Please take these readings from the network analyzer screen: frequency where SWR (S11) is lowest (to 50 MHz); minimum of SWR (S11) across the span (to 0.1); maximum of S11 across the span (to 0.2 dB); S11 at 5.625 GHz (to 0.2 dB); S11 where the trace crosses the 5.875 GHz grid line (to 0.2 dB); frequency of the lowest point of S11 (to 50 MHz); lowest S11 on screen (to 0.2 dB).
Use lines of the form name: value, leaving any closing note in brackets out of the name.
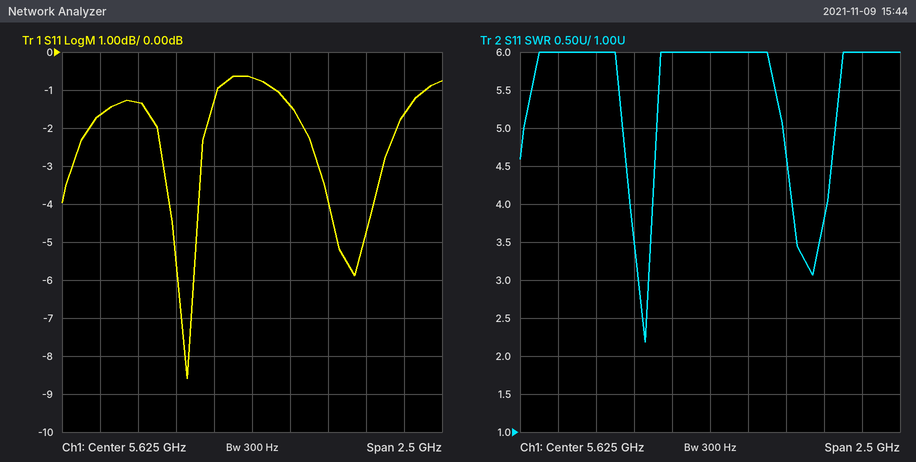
frequency where SWR (S11) is lowest: 5.20 GHz
minimum of SWR (S11) across the span: 2.2
maximum of S11 across the span: -0.6 dB
S11 at 5.625 GHz: -0.6 dB
S11 where the trace crosses the 5.875 GHz grid line: -1.4 dB
frequency of the lowest point of S11: 5.20 GHz
lowest S11 on screen: -8.6 dB
